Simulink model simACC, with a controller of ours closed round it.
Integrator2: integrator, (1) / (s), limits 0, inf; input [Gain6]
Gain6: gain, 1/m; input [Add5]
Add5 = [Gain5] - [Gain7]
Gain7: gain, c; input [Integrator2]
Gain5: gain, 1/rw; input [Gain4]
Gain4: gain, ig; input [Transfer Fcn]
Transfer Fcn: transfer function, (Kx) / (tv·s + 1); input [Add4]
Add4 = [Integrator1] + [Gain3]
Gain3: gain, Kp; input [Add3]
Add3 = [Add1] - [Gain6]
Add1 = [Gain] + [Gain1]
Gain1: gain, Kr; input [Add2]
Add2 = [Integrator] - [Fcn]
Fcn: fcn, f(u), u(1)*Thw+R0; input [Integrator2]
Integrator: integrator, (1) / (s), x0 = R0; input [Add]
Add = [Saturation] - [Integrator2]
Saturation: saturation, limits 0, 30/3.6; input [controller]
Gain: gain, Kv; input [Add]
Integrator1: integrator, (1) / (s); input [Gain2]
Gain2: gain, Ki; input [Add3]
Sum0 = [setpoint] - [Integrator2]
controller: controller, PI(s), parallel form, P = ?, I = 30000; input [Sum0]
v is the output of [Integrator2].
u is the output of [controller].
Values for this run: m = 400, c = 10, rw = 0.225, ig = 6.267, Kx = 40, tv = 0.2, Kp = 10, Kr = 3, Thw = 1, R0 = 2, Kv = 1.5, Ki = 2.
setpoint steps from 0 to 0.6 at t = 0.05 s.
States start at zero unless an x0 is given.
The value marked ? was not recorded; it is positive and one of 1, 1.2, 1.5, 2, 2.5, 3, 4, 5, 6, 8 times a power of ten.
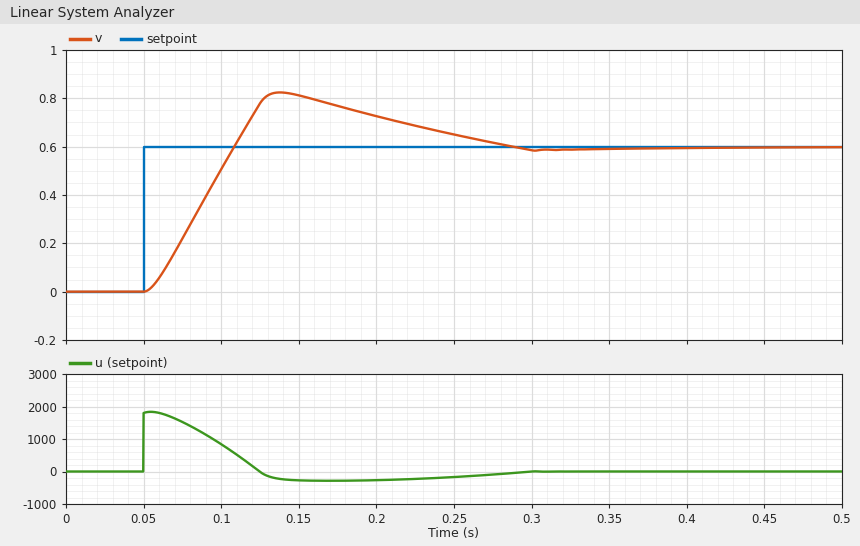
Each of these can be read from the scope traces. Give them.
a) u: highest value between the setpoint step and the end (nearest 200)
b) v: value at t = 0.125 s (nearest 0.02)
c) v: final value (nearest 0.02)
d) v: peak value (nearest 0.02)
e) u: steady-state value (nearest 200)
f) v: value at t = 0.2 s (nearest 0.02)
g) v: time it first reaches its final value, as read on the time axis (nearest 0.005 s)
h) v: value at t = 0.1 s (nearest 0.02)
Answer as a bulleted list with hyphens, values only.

- 1800
- 0.78
- 0.60
- 0.82
- 0
- 0.72
- 0.110 s
- 0.50
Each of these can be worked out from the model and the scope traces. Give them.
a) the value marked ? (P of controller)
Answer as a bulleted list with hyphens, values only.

- 3000
